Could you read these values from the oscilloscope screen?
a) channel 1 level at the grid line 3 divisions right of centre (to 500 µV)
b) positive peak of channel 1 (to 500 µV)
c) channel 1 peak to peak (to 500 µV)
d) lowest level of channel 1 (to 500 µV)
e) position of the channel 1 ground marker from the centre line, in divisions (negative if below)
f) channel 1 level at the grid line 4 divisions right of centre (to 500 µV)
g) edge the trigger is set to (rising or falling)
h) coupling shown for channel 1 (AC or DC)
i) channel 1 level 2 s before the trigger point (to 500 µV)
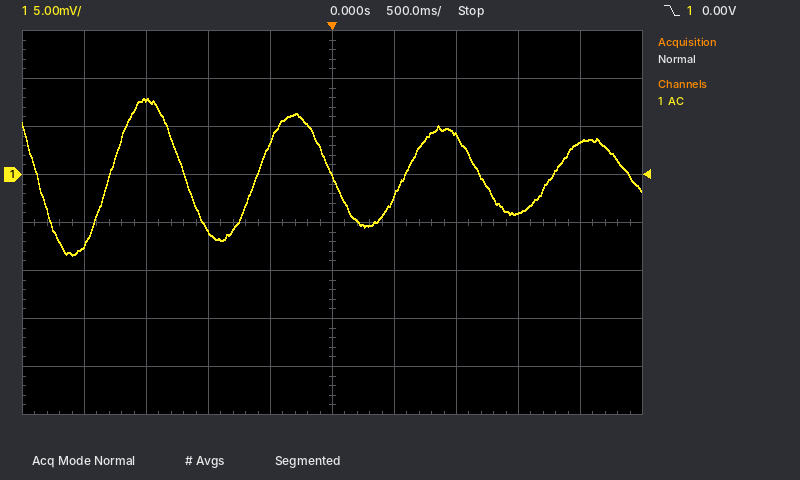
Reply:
-4.0 mV
8.0 mV
16.5 mV
-8.5 mV
+1.0 div
3.5 mV
falling
AC
-7.5 mV
